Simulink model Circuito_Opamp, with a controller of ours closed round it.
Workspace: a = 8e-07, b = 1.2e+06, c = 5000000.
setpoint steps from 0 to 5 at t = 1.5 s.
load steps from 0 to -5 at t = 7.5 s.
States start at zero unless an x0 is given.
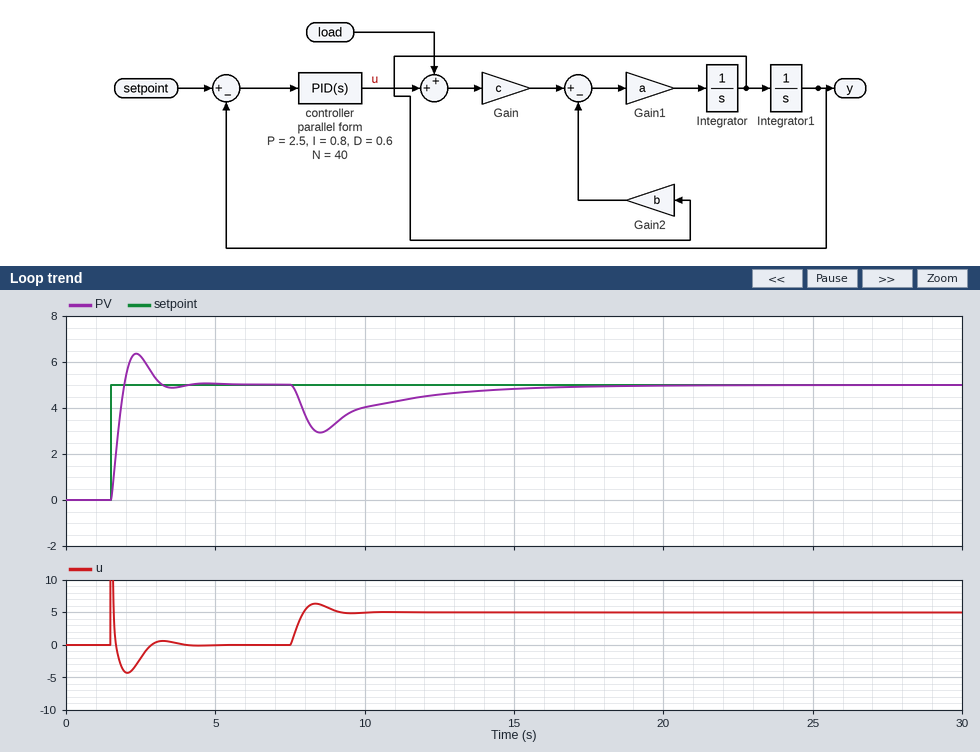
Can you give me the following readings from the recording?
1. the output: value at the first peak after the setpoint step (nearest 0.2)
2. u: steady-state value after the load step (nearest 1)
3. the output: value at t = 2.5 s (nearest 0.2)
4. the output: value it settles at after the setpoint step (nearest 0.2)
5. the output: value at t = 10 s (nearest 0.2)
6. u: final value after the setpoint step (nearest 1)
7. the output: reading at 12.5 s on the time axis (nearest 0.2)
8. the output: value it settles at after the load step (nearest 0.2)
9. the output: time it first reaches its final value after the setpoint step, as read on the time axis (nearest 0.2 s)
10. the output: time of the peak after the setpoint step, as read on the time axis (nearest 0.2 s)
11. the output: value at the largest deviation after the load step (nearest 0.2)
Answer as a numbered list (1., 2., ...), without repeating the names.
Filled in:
1. 6.4
2. 5
3. 6.2
4. 5.0
5. 4.0
6. 0
7. 4.6
8. 5.0
9. 2.0 s
10. 2.4 s
11. 3.0
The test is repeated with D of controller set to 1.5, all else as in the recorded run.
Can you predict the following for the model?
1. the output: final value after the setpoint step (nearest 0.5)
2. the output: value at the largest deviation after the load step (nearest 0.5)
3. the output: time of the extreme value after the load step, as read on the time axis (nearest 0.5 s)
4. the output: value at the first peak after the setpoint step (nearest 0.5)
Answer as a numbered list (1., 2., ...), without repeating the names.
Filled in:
1. 5.0
2. 3.5
3. 9.0 s
4. 5.5
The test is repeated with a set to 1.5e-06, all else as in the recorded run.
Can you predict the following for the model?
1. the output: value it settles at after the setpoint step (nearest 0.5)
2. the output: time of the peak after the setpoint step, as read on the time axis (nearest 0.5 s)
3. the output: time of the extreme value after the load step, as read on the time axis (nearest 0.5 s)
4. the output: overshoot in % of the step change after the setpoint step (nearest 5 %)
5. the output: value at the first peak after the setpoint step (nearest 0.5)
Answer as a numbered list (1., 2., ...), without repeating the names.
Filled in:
1. 5.0
2. 2.0 s
3. 8.5 s
4. 15 %
5. 5.5
